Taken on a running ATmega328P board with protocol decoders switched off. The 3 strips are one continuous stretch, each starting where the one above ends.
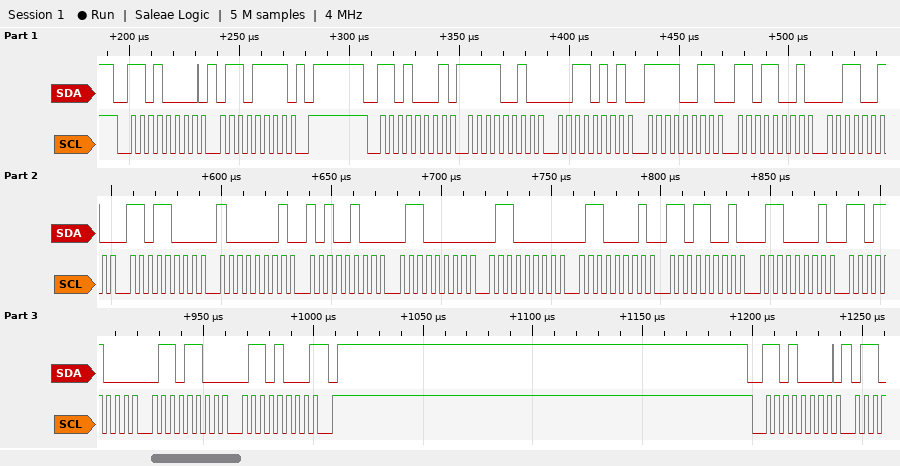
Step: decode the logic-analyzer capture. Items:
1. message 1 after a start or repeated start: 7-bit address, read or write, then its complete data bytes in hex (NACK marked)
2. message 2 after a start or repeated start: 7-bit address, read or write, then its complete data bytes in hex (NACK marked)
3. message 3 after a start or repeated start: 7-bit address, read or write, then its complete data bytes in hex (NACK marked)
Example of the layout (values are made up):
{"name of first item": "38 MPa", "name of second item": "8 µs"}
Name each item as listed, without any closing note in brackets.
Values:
{"message 1 after a start or repeated start: 7-bit address, read or write, then its complete data bytes in hex": "0x68 write: 6F", "message 2 after a start or repeated start: 7-bit address, read or write, then its complete data bytes in hex": "0x68 read: F2 35 F3 D9 32 D8 81 A4 60 60 61 D9 61 D8 6C 68 NACK", "message 3 after a start or repeated start: 7-bit address, read or write, then its complete data bytes in hex": "0x68 write"}
